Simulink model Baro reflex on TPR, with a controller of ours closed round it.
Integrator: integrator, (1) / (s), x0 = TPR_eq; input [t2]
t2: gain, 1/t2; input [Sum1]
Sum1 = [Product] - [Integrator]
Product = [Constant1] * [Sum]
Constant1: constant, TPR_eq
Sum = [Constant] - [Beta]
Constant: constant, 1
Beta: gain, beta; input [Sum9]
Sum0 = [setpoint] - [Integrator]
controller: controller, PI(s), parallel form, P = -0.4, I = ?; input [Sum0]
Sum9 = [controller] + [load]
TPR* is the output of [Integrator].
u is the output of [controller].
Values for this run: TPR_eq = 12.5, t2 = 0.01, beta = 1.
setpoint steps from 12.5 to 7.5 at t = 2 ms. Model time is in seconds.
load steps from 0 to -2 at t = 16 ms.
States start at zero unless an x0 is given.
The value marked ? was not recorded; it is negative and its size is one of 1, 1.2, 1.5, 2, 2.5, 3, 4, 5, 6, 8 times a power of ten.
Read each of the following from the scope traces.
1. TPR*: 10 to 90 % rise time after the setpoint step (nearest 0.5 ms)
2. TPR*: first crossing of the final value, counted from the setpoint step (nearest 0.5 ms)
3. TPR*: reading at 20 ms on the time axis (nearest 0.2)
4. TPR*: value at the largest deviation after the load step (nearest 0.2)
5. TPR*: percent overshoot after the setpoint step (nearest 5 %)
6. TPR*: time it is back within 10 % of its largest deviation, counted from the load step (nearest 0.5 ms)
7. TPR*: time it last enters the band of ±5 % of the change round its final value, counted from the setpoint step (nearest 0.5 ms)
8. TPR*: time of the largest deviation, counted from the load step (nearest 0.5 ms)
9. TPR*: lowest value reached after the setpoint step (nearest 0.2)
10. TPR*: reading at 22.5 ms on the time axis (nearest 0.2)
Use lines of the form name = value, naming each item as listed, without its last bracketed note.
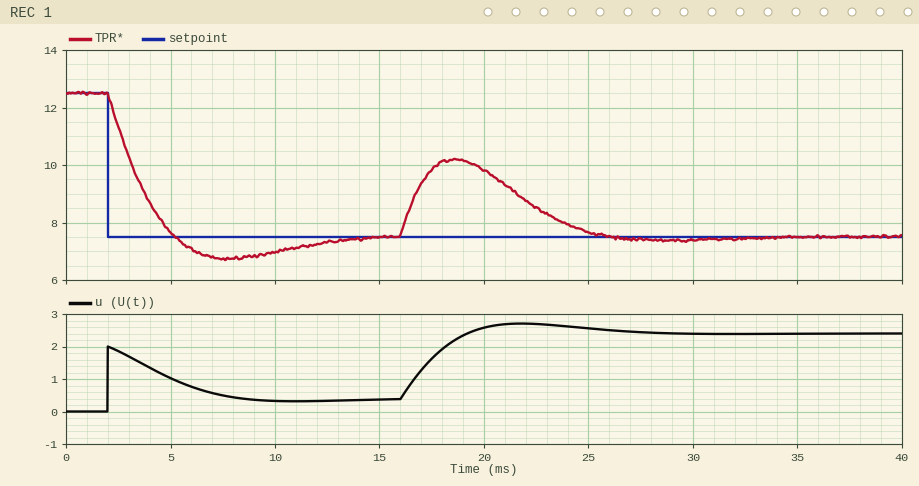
TPR*: 10 to 90 % rise time after the setpoint step = 2.5 ms
TPR*: first crossing of the final value, counted from the setpoint step = 3.0 ms
TPR*: reading at 20 ms on the time axis = 9.8
TPR*: value at the largest deviation after the load step = 10.2
TPR*: percent overshoot after the setpoint step = 15 %
TPR*: time it is back within 10 % of its largest deviation, counted from the load step = 8.5 ms
TPR*: time it last enters the band of ±5 % of the change round its final value, counted from the setpoint step = 10.0 ms
TPR*: time of the largest deviation, counted from the load step = 2.5 ms
TPR*: lowest value reached after the setpoint step = 6.8
TPR*: reading at 22.5 ms on the time axis = 8.6
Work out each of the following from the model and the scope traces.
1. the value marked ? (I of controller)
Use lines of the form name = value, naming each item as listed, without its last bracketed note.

the value marked ? = -150
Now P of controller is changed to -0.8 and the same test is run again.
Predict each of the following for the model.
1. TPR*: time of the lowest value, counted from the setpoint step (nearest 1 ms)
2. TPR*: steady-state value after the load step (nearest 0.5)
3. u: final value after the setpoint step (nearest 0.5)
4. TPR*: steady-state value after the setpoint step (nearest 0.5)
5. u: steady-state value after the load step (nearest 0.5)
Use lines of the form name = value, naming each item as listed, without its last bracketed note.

TPR*: time of the lowest value, counted from the setpoint step = 5 ms
TPR*: steady-state value after the load step = 7.5
u: final value after the setpoint step = 0.5
TPR*: steady-state value after the setpoint step = 7.5
u: steady-state value after the load step = 2.5
